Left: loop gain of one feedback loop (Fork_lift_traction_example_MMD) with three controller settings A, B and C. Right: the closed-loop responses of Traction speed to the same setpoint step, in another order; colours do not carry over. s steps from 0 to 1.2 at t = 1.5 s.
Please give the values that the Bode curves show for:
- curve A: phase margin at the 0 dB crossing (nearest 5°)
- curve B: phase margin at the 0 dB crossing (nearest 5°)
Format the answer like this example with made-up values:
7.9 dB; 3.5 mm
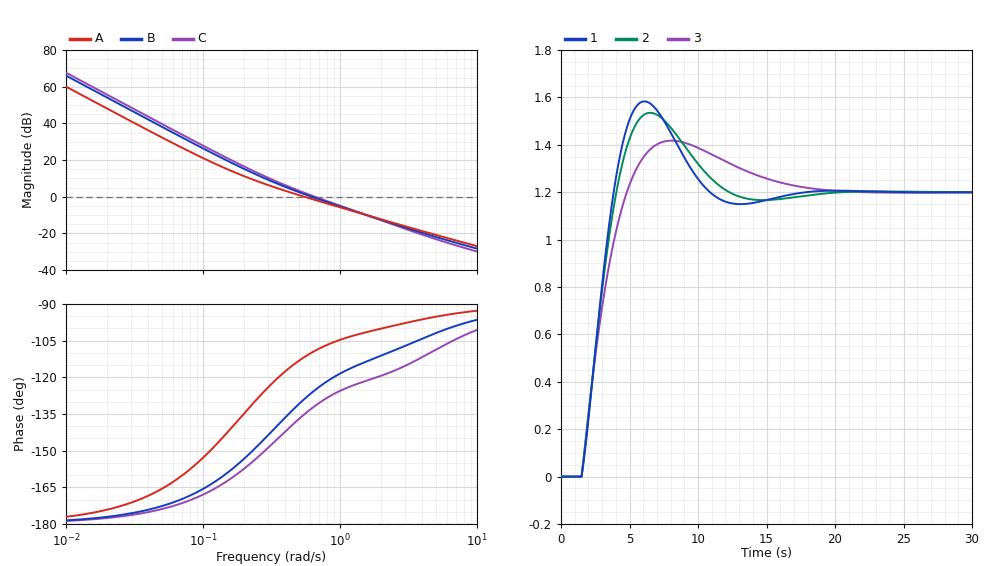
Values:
70°; 55°
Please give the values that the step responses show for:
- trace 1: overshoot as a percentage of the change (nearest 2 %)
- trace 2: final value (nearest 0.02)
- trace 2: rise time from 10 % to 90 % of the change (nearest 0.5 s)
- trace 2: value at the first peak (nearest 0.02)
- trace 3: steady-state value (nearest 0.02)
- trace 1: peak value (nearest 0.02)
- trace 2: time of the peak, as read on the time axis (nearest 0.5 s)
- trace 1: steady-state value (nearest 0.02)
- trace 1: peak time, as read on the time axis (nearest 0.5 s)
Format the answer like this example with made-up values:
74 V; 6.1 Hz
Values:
32 %; 1.20; 2.0 s; 1.54; 1.20; 1.58; 6.5 s; 1.20; 6.0 s
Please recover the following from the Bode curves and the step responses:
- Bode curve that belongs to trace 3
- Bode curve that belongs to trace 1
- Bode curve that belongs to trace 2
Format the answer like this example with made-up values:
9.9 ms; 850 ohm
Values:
A; C; B
